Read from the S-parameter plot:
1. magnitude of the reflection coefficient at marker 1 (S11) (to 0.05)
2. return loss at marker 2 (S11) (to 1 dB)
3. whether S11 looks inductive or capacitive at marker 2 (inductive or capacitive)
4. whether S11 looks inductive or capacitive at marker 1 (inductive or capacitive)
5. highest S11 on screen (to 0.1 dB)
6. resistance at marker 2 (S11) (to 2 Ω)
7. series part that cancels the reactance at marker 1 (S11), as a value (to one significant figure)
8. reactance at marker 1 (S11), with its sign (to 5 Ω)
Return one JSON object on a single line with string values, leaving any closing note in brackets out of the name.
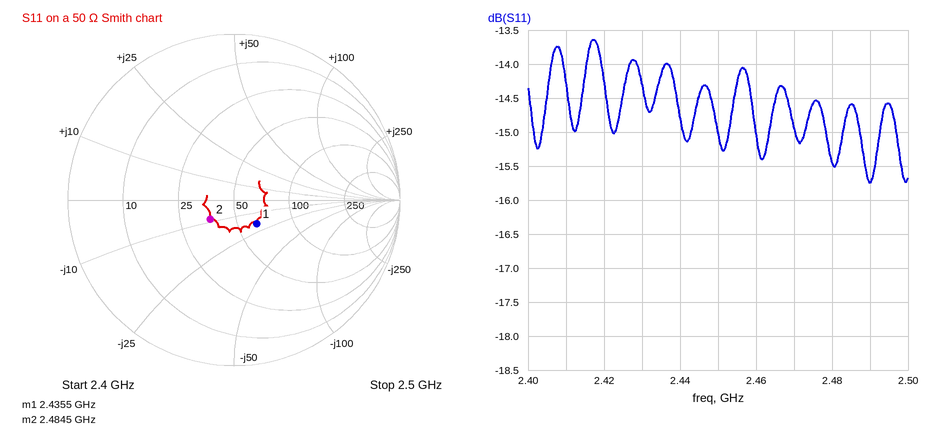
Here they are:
{"magnitude of the reflection coefficient at marker 1 (S11)": "0.20", "return loss at marker 2 (S11)": "15 dB", "whether S11 looks inductive or capacitive at marker 2": "capacitive", "whether S11 looks inductive or capacitive at marker 1": "capacitive", "highest S11 on screen": "-13.6 dB", "resistance at marker 2 (S11)": "36 Ω", "series part that cancels the reactance at marker 1 (S11), as a value": "1 nH", "reactance at marker 1 (S11), with its sign": "-20 Ω"}
